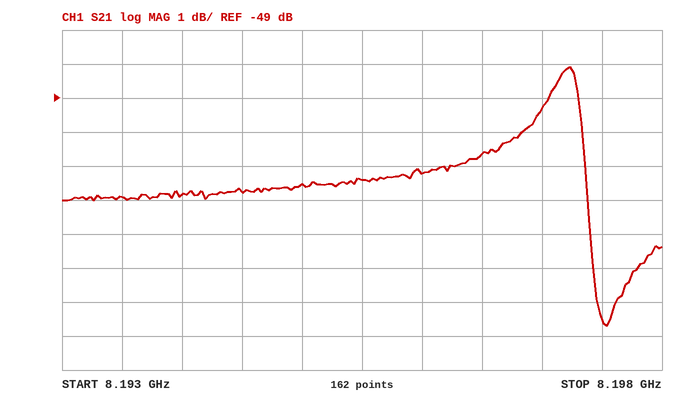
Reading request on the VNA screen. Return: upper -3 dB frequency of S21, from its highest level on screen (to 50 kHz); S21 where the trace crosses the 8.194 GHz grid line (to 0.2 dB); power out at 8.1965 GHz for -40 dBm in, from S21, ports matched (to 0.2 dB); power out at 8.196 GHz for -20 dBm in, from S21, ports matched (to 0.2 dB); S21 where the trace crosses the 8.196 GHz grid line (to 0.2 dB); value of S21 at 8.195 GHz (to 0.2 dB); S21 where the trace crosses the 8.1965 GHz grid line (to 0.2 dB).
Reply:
8.19735 GHz
-51.8 dB
-90.6 dBm
-71.2 dBm
-51.2 dB
-51.6 dB
-50.6 dB
